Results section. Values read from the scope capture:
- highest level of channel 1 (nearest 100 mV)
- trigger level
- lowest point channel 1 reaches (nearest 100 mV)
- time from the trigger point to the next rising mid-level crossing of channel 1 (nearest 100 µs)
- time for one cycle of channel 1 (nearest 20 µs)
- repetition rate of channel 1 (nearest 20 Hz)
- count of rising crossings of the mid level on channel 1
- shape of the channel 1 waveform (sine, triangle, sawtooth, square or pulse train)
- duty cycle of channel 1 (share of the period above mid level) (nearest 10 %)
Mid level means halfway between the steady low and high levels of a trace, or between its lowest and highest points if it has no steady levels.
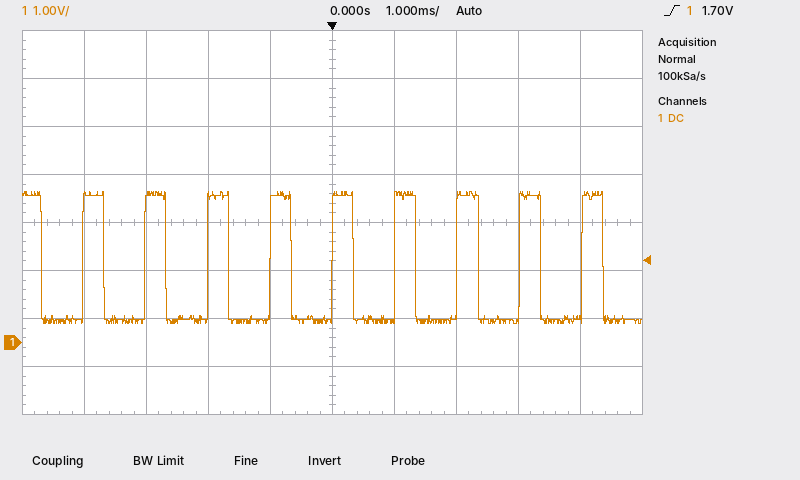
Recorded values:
3.1 V
1.70 V
400 mV
1.0 ms
1.00 ms
1.00 kHz
9
pulse train
30 %
